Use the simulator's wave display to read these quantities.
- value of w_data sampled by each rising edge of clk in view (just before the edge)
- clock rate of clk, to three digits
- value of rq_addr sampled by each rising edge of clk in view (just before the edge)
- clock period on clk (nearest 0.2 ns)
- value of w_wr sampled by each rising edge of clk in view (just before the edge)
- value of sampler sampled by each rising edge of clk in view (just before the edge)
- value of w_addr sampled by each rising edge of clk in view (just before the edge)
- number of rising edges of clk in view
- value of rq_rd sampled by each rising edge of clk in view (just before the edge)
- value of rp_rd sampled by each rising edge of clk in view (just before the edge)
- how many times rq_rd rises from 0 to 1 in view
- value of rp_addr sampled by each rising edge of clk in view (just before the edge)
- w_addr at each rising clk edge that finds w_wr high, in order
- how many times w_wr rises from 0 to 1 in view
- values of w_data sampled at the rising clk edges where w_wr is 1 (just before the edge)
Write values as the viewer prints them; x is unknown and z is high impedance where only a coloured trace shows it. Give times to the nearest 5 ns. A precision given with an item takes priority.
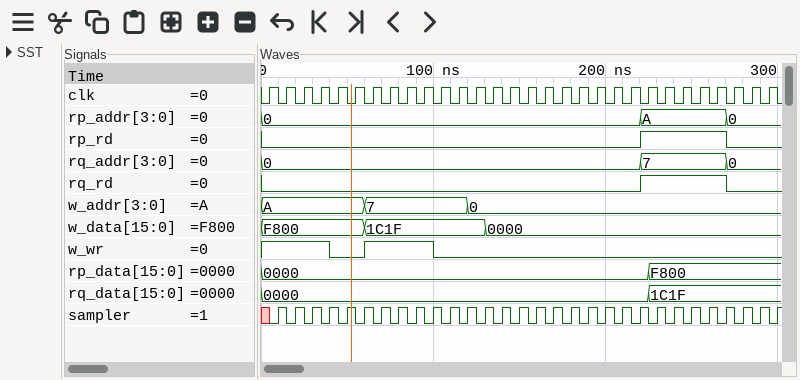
F800, F800, F800, F800, F800, F800, 1C1F, 1C1F, 1C1F, 1C1F, 1C1F, 1C1F, 1C1F, 0000, 0000, 0000, 0000, 0000, 0000, 0000, 0000, 0000, 0000, 0000, 0000, 0000, 0000, 0000, 0000, 0000
100 MHz
0, 0, 0, 0, 0, 0, 0, 0, 0, 0, 0, 0, 0, 0, 0, 0, 0, 0, 0, 0, 0, 0, 7, 7, 7, 7, 7, 0, 0, 0
10 ns
1 1 1 1 0 0 1 1 1 1 0 0 0 0 0 0 0 0 0 0 0 0 0 0 0 0 0 0 0 0
x 1 1 1 1 1 1 1 1 1 1 1 1 1 1 1 1 1 1 1 1 1 1 1 1 1 1 1 1 1
A, A, A, A, A, A, 7, 7, 7, 7, 7, 7, 0, 0, 0, 0, 0, 0, 0, 0, 0, 0, 0, 0, 0, 0, 0, 0, 0, 0
30
0 0 0 0 0 0 0 0 0 0 0 0 0 0 0 0 0 0 0 0 0 0 1 1 1 1 1 0 0 0
0 0 0 0 0 0 0 0 0 0 0 0 0 0 0 0 0 0 0 0 0 0 1 1 1 1 1 0 0 0
1
0, 0, 0, 0, 0, 0, 0, 0, 0, 0, 0, 0, 0, 0, 0, 0, 0, 0, 0, 0, 0, 0, A, A, A, A, A, 0, 0, 0
A, A, A, A, 7, 7, 7, 7
1
F800, F800, F800, F800, 1C1F, 1C1F, 1C1F, 1C1F
